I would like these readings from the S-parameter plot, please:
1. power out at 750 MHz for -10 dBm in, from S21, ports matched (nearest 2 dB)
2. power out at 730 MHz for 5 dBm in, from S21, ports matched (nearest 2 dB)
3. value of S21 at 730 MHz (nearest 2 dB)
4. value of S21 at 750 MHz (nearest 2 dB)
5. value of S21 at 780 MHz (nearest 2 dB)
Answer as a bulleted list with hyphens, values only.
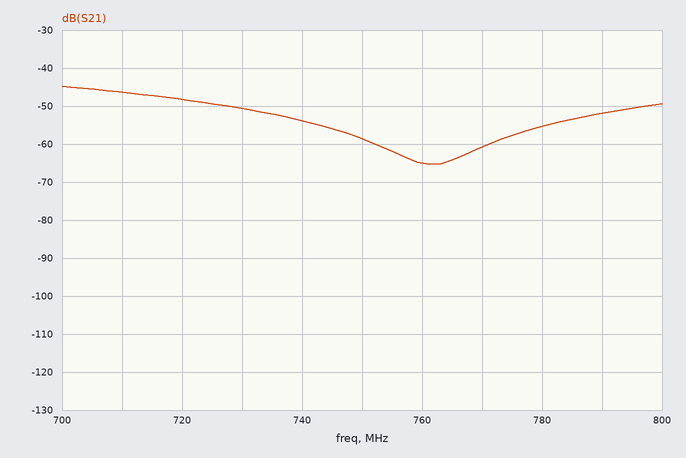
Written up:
- -68 dBm
- -46 dBm
- -50 dB
- -58 dB
- -56 dB
